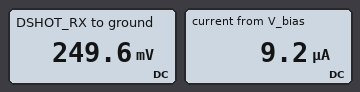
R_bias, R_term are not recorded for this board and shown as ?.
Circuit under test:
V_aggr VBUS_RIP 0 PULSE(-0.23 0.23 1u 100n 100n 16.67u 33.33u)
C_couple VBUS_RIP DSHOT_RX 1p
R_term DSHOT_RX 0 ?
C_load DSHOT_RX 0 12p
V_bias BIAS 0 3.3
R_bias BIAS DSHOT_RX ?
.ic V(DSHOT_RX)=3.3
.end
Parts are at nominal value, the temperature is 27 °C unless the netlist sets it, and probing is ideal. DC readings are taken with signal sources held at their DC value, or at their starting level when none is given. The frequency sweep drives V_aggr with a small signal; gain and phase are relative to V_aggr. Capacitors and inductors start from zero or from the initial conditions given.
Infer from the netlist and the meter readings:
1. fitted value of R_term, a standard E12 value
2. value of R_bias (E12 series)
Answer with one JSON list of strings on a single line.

["27 kΩ", "330 kΩ"]
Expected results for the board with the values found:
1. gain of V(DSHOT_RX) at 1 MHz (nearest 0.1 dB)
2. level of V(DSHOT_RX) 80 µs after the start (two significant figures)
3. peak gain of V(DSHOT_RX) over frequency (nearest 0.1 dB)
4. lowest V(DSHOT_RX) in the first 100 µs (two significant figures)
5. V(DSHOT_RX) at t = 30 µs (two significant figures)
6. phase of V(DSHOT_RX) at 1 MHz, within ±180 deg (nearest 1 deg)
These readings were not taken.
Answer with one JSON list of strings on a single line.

["-23.2 dB", "250 mV", "-22.3 dB", "220 mV", "250 mV", "26 deg"]
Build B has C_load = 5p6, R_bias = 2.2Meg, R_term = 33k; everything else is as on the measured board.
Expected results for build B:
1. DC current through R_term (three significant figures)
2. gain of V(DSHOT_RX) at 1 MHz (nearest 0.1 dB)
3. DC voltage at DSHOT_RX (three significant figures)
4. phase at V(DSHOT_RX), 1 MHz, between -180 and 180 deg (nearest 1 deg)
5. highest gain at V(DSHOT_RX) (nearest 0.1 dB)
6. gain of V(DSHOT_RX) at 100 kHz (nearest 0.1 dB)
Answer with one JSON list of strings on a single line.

["1.48 µA", "-18.3 dB", "48.8 mV", "37 deg", "-16.4 dB", "-33.9 dB"]
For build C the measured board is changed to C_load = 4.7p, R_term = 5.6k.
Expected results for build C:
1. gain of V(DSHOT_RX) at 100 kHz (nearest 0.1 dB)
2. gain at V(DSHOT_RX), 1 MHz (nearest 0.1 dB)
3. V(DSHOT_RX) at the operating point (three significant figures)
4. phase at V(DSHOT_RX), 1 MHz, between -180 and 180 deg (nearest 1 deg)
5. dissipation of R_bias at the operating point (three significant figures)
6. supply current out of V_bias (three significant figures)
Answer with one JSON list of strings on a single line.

["-49.2 dB", "-29.4 dB", "55.1 mV", "79 deg", "31.9 µW", "9.83 µA"]
